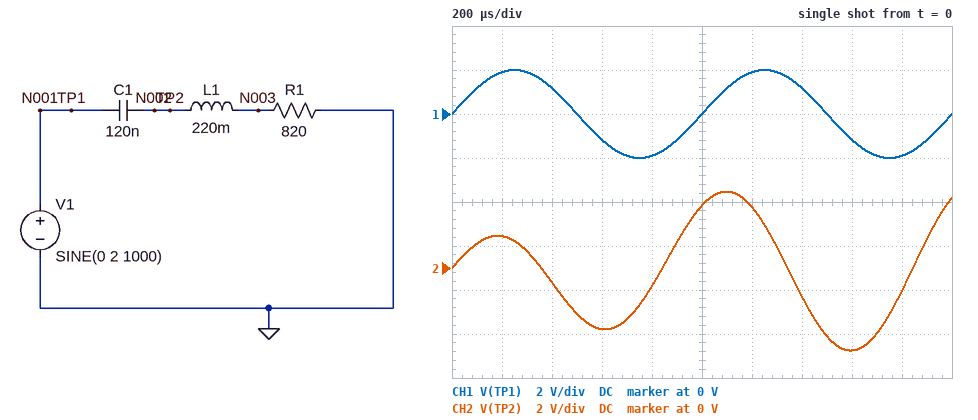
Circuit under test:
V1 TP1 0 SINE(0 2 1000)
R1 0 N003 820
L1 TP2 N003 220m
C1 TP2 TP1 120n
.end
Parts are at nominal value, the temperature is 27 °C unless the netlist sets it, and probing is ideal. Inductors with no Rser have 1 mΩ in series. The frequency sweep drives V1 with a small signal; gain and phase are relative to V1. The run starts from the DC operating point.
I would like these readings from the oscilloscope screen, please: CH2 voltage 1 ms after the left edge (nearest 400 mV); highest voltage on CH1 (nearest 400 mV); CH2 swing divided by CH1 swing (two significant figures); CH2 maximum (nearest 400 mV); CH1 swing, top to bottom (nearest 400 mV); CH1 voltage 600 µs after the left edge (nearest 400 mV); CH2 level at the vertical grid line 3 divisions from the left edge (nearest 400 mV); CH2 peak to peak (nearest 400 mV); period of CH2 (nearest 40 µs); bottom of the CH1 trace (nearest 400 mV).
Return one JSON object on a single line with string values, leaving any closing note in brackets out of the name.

{"CH2 voltage 1 ms after the left edge": "2.8 V", "highest voltage on CH1": "2.0 V", "CH2 swing divided by CH1 swing": "1.8", "CH2 maximum": "3.6 V", "CH1 swing, top to bottom": "4.0 V", "CH1 voltage 600 µs after the left edge": "-1.2 V", "CH2 level at the vertical grid line 3 divisions from the left edge": "-2.8 V", "CH2 peak to peak": "7.2 V", "period of CH2": "1.00 ms", "bottom of the CH1 trace": "-2.0 V"}
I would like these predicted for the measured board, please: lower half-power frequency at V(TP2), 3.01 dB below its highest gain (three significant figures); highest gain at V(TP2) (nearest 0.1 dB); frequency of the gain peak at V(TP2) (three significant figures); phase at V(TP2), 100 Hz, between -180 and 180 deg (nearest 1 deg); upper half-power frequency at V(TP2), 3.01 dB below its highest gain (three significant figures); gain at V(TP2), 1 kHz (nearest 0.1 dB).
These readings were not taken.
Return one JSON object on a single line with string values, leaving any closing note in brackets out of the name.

{"lower half-power frequency at V(TP2), 3.01 dB below its highest gain": "802 Hz", "highest gain at V(TP2)": "5.9 dB", "frequency of the gain peak at V(TP2)": "1.05 kHz", "phase at V(TP2), 100 Hz, between -180 and 180 deg": "96 deg", "upper half-power frequency at V(TP2), 3.01 dB below its highest gain": "1.71 kHz", "gain at V(TP2), 1 kHz": "5.8 dB"}
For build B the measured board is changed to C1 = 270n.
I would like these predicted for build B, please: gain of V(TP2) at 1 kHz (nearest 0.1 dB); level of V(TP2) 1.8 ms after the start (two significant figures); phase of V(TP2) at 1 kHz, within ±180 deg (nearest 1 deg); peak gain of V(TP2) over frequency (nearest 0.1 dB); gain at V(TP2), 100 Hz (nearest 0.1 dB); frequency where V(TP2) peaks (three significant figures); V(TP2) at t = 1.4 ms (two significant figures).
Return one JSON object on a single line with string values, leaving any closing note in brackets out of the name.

{"gain of V(TP2) at 1 kHz": "3.0 dB", "level of V(TP2) 1.8 ms after the start": "-2.4 V", "phase of V(TP2) at 1 kHz, within ±180 deg": "15 deg", "peak gain of V(TP2) over frequency": "3.8 dB", "gain at V(TP2), 100 Hz": "-16.9 dB", "frequency where V(TP2) peaks": "749 Hz", "V(TP2) at t = 1.4 ms": "1.1 V"}
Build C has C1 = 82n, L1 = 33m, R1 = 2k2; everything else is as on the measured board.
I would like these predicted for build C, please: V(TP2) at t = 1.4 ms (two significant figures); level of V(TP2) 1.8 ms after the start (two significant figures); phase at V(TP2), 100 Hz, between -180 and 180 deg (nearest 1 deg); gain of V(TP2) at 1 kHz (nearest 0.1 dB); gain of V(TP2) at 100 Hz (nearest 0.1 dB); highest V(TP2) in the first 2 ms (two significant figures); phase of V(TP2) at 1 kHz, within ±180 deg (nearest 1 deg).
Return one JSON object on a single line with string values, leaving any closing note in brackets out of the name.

{"V(TP2) at t = 1.4 ms": "-210 mV", "level of V(TP2) 1.8 ms after the start": "-750 mV", "phase at V(TP2), 100 Hz, between -180 and 180 deg": "84 deg", "gain of V(TP2) at 1 kHz": "-2.1 dB", "gain of V(TP2) at 100 Hz": "-19.0 dB", "highest V(TP2) in the first 2 ms": "1.6 V", "phase of V(TP2) at 1 kHz, within ±180 deg": "44 deg"}
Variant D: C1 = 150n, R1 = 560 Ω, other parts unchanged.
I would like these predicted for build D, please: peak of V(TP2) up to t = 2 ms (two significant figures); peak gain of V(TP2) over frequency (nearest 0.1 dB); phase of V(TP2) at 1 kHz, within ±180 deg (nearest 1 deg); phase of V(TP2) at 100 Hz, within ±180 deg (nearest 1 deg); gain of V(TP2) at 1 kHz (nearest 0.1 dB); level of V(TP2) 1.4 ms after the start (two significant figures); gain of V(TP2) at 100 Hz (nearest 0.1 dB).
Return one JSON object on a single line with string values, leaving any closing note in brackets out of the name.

{"peak of V(TP2) up to t = 2 ms": "4.1 V", "peak gain of V(TP2) over frequency": "7.7 dB", "phase of V(TP2) at 1 kHz, within ±180 deg": "38 deg", "phase of V(TP2) at 100 Hz, within ±180 deg": "101 deg", "gain of V(TP2) at 1 kHz": "7.3 dB", "level of V(TP2) 1.4 ms after the start": "-750 mV", "gain of V(TP2) at 100 Hz": "-25.2 dB"}
